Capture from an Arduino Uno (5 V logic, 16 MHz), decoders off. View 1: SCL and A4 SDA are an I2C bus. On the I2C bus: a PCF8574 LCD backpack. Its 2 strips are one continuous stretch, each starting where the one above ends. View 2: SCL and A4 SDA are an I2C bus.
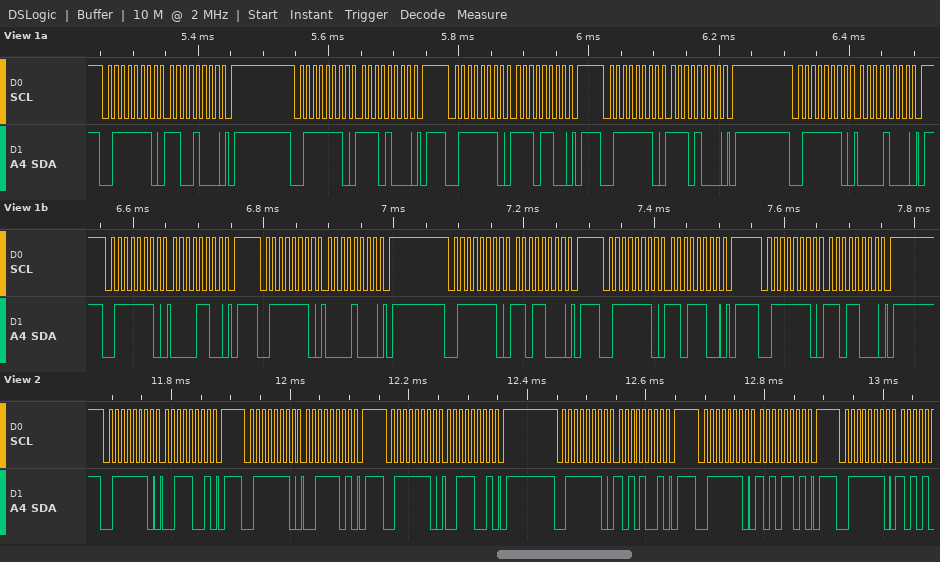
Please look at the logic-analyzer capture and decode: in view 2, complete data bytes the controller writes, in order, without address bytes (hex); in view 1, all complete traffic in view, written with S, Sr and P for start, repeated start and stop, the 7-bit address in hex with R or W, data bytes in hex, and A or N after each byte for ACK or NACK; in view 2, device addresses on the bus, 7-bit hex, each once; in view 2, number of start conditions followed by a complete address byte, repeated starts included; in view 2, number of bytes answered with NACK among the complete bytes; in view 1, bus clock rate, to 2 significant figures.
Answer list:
39 3D 39 A9 AD
S 3FW A C8 A P S 3FW A E8 A P S 3FW A EC A P S 3FW A E8 A P S 3FW A 08 A P S 3FW A 0C A P S 3FW A 08 A P S 3FW A D8 A P S 3FW A DC A P S 3FW A D8 A P
0x3F
6
0
100 kHz
